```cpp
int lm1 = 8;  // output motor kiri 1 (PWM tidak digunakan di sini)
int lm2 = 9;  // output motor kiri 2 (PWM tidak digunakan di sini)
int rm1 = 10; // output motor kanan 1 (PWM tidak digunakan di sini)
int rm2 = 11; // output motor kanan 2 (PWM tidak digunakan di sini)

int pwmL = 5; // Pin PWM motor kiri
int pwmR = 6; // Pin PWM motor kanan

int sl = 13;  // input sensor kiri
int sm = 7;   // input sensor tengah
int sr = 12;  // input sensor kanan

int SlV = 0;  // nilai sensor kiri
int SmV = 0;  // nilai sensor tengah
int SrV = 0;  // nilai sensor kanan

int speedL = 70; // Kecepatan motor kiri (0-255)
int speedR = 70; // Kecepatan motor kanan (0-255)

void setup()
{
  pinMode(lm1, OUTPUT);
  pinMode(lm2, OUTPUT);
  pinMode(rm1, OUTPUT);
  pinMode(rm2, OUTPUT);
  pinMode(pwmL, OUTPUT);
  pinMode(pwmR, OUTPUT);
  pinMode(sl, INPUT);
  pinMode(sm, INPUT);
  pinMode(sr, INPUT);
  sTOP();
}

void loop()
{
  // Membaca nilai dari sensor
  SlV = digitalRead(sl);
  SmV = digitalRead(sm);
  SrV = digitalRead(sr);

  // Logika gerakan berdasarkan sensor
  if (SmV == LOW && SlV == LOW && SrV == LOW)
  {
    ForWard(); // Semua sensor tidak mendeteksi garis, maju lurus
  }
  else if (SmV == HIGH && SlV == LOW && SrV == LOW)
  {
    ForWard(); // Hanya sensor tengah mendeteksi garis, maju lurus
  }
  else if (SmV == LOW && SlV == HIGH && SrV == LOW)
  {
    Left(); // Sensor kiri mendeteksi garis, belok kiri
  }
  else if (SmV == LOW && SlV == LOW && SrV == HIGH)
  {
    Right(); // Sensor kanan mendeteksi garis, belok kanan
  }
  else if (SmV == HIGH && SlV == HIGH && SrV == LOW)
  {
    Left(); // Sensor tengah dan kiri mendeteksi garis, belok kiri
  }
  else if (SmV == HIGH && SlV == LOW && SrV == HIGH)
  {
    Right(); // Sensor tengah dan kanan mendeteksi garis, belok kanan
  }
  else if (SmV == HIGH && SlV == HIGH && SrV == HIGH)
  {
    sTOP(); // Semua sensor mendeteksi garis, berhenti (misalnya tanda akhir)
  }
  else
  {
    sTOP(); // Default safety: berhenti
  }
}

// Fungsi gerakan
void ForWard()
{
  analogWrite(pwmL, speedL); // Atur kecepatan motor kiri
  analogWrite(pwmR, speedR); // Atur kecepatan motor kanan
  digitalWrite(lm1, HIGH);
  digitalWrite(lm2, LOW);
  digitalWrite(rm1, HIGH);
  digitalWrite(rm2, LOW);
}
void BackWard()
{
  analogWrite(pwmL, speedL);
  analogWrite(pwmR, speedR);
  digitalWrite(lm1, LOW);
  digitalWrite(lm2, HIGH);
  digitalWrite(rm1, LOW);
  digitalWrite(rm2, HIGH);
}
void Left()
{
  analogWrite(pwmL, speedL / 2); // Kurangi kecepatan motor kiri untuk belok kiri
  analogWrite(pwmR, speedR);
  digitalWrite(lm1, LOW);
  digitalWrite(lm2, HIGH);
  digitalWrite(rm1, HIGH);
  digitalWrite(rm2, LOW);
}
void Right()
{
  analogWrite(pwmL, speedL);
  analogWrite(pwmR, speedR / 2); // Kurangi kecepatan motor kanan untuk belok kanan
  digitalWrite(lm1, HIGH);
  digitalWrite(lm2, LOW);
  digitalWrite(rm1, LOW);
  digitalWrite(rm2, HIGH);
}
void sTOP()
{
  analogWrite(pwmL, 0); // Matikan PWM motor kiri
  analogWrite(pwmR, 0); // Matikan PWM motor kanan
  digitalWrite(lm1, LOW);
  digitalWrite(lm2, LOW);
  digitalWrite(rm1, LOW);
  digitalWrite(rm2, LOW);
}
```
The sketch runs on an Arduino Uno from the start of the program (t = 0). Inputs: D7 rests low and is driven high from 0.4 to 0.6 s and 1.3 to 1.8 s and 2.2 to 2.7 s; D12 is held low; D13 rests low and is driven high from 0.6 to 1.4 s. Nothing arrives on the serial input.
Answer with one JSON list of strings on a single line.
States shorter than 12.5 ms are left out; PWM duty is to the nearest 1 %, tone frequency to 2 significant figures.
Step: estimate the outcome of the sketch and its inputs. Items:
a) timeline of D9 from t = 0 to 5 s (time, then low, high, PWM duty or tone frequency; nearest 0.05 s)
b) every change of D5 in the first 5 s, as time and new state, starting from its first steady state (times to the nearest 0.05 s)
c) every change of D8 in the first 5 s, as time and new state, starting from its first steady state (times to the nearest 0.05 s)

["0 s low; 0.6 s high; 1.4 s low", "0 s PWM 28 %; 0.6 s PWM 14 %; 1.4 s PWM 28 %", "0 s high; 0.6 s low; 1.4 s high"]
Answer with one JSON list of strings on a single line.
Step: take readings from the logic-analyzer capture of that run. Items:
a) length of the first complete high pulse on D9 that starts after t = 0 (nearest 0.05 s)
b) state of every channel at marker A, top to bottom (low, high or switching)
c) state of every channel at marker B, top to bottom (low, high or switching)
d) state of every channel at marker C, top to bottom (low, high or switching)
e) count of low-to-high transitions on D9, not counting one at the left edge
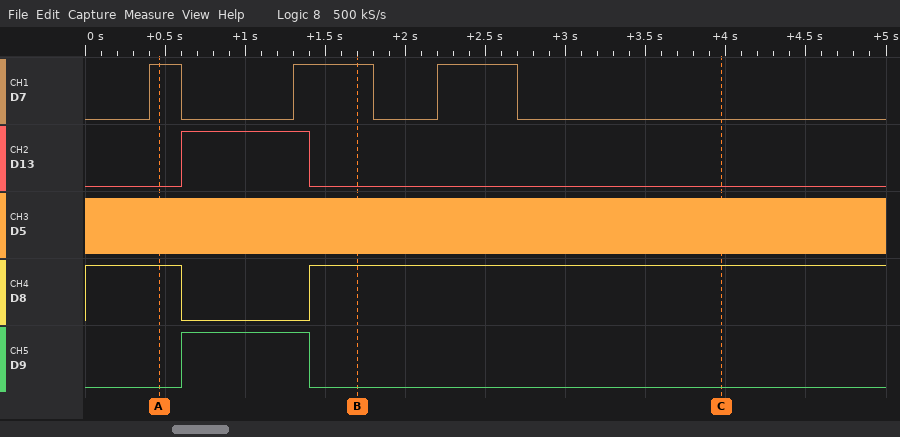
["0.80 s", "D7 high, D13 low, D5 switching, D8 high, D9 low", "D7 high, D13 low, D5 switching, D8 high, D9 low", "D7 low, D13 low, D5 switching, D8 high, D9 low", "1"]
